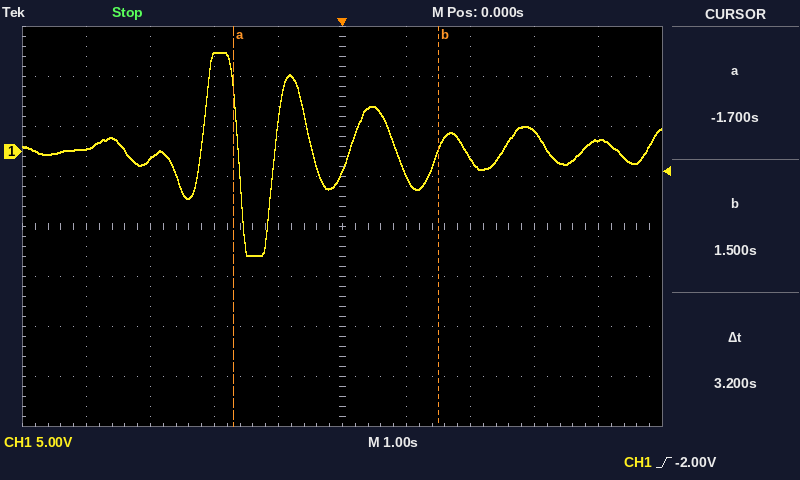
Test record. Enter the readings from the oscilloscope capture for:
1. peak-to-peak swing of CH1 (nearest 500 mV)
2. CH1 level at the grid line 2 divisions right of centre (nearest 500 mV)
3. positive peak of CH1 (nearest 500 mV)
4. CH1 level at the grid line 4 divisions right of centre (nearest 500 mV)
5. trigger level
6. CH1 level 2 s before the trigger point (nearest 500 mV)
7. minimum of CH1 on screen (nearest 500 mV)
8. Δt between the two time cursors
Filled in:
20.5 V
-500 mV
10.0 V
1.0 V
-2.00 V
9.5 V
-10.5 V
3.2 s
